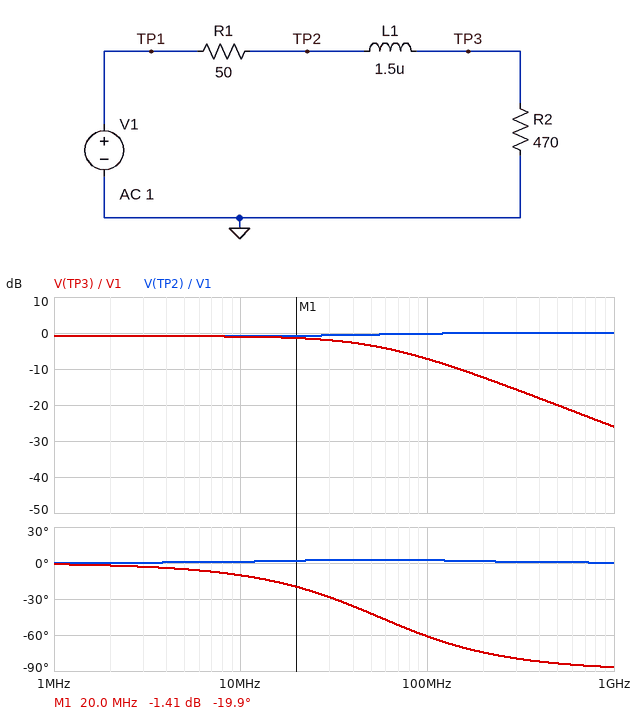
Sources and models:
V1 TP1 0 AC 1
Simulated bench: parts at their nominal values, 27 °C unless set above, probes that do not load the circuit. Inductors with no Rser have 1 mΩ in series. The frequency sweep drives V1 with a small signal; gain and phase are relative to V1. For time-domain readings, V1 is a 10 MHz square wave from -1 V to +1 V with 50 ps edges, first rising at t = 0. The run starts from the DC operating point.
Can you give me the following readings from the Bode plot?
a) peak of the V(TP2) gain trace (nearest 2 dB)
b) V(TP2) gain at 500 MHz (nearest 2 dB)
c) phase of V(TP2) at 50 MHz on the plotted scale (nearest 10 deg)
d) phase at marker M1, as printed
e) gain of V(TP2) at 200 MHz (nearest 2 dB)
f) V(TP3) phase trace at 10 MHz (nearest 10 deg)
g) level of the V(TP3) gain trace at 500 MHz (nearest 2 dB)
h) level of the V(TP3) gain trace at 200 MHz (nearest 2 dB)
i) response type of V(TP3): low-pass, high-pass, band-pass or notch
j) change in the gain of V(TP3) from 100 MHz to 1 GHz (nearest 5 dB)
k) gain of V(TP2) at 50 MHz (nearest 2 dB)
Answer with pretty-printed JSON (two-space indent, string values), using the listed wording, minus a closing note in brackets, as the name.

{
  "peak of the V(TP2) gain trace": "0 dB",
  "V(TP2) gain at 500 MHz": "0 dB",
  "phase of V(TP2) at 50 MHz on the plotted scale": "0 deg",
  "phase at marker M1, as printed": "-19.9 deg",
  "gain of V(TP2) at 200 MHz": "0 dB",
  "V(TP3) phase trace at 10 MHz": "-10 deg",
  "level of the V(TP3) gain trace at 500 MHz": "-20 dB",
  "level of the V(TP3) gain trace at 200 MHz": "-12 dB",
  "response type of V(TP3): low-pass, high-pass, band-pass or notch": "low-pass",
  "change in the gain of V(TP3) from 100 MHz to 1 GHz": "-20 dB",
  "gain of V(TP2) at 50 MHz": "0 dB"
}
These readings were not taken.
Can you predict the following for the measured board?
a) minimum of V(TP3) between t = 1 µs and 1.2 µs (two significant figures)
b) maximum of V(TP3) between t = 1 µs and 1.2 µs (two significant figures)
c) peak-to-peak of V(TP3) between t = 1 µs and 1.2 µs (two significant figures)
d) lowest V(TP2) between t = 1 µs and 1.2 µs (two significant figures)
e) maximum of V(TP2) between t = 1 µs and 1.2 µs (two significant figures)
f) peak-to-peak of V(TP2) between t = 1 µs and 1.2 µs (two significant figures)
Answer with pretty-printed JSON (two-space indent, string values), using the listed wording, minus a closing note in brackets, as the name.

{
  "minimum of V(TP3) between t = 1 µs and 1.2 µs": "-900 mV",
  "maximum of V(TP3) between t = 1 µs and 1.2 µs": "900 mV",
  "peak-to-peak of V(TP3) between t = 1 µs and 1.2 µs": "1.8 V",
  "lowest V(TP2) between t = 1 µs and 1.2 µs": "-1.1 V",
  "maximum of V(TP2) between t = 1 µs and 1.2 µs": "1.1 V",
  "peak-to-peak of V(TP2) between t = 1 µs and 1.2 µs": "2.2 V"
}
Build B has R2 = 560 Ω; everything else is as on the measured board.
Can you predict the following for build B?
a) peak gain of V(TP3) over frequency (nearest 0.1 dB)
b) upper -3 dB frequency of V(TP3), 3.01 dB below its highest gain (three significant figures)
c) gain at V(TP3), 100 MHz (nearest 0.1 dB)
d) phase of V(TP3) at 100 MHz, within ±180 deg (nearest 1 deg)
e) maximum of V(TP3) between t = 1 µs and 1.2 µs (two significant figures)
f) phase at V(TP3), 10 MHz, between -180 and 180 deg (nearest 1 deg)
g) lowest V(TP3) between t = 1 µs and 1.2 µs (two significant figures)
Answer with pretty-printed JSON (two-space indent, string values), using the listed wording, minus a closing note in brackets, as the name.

{
  "peak gain of V(TP3) over frequency": "-0.7 dB",
  "upper -3 dB frequency of V(TP3), 3.01 dB below its highest gain": "64.7 MHz",
  "gain at V(TP3), 100 MHz": "-6.0 dB",
  "phase of V(TP3) at 100 MHz, within ±180 deg": "-57 deg",
  "maximum of V(TP3) between t = 1 µs and 1.2 µs": "920 mV",
  "phase at V(TP3), 10 MHz, between -180 and 180 deg": "-9 deg",
  "lowest V(TP3) between t = 1 µs and 1.2 µs": "-920 mV"
}
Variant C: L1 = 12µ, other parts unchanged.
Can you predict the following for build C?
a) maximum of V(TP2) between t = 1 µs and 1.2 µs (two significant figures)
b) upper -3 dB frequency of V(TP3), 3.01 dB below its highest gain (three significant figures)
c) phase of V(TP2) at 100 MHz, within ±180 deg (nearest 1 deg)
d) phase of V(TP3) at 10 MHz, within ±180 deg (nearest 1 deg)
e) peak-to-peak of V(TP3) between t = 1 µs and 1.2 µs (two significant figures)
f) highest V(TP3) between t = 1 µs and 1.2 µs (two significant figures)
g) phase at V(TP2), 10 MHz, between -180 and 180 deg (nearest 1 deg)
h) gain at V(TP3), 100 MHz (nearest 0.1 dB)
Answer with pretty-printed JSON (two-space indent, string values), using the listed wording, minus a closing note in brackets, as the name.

{
  "maximum of V(TP2) between t = 1 µs and 1.2 µs": "1.1 V",
  "upper -3 dB frequency of V(TP3), 3.01 dB below its highest gain": "6.90 MHz",
  "phase of V(TP2) at 100 MHz, within ±180 deg": "0 deg",
  "phase of V(TP3) at 10 MHz, within ±180 deg": "-55 deg",
  "peak-to-peak of V(TP3) between t = 1 µs and 1.2 µs": "1.4 V",
  "highest V(TP3) between t = 1 µs and 1.2 µs": "720 mV",
  "phase at V(TP2), 10 MHz, between -180 and 180 deg": "3 deg",
  "gain at V(TP3), 100 MHz": "-24.1 dB"
}
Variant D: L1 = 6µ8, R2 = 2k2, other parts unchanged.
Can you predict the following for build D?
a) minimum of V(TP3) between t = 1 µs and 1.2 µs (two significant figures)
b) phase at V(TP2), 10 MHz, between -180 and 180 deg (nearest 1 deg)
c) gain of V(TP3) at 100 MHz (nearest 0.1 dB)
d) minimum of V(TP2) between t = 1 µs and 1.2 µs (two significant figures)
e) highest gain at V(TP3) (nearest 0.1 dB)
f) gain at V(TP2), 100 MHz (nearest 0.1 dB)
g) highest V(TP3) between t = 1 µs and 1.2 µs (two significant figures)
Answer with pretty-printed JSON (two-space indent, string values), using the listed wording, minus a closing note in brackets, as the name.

{
  "minimum of V(TP3) between t = 1 µs and 1.2 µs": "-980 mV",
  "phase at V(TP2), 10 MHz, between -180 and 180 deg": "0 deg",
  "gain of V(TP3) at 100 MHz": "-6.8 dB",
  "minimum of V(TP2) between t = 1 µs and 1.2 µs": "-1.0 V",
  "highest gain at V(TP3)": "-0.2 dB",
  "gain at V(TP2), 100 MHz": "0 dB",
  "highest V(TP3) between t = 1 µs and 1.2 µs": "980 mV"
}
